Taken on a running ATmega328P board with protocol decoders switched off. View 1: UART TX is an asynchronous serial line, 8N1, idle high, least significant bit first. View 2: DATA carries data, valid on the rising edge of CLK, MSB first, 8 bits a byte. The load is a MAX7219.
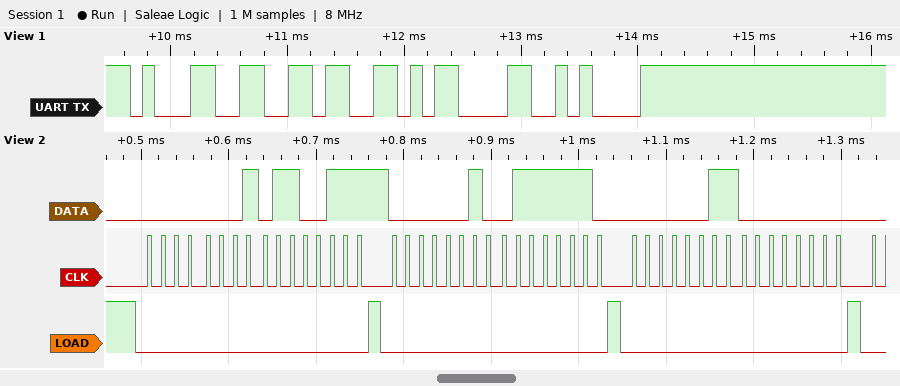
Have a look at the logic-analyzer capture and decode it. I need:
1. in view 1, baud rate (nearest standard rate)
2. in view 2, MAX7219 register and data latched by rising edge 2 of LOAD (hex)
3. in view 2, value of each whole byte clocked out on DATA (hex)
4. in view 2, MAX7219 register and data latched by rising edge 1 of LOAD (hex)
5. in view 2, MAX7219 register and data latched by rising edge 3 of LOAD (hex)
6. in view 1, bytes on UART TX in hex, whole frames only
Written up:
9600 baud
register 0x2, data 0x7E
01 67 02 7E 03 00
register 0x1, data 0x67
register 0x3, data 0x00
0x31 0x36 0x0D 0x0A
